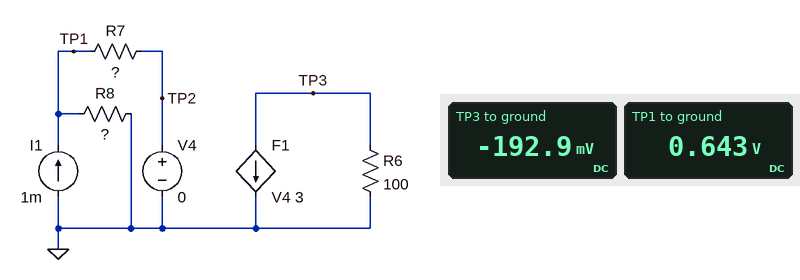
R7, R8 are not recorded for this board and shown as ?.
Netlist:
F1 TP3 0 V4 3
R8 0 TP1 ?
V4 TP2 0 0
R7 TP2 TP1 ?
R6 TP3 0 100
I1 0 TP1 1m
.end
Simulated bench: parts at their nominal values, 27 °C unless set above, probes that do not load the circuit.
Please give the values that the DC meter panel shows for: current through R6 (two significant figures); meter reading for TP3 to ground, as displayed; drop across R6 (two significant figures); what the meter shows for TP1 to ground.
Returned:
1.9 mA
-192.9 mV
190 mV
0.643 V
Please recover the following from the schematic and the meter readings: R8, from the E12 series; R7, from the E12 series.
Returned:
1.8 kΩ
1 kΩ
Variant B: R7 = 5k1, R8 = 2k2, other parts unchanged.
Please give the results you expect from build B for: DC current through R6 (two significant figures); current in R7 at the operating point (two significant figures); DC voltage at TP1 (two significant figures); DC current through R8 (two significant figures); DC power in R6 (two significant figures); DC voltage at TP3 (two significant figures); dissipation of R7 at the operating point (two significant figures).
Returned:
900 µA
300 µA
1.5 V
700 µA
82 µW
-90 mV
460 µW
